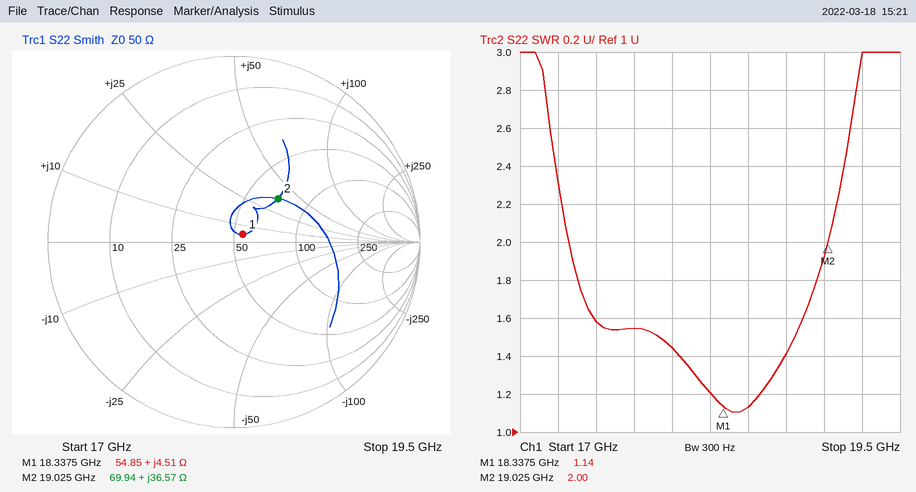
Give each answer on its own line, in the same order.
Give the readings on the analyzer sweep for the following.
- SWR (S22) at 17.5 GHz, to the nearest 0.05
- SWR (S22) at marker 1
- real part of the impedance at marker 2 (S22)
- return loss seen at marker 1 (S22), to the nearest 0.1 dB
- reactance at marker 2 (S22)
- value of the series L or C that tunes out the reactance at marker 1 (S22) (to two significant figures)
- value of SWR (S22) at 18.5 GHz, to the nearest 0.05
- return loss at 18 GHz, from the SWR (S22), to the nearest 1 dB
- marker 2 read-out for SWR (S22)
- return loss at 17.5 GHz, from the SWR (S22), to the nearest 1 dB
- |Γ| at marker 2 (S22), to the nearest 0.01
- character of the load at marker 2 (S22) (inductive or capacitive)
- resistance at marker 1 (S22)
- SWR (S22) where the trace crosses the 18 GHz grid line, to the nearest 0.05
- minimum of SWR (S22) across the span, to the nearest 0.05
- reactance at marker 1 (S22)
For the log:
1.60
1.14
69.94 Ω
24.0 dB
+36.57 Ω
1.9 pF
1.15
15 dB
2.00
13 dB
0.33
inductive
54.85 Ω
1.45
1.10
+4.51 Ω
